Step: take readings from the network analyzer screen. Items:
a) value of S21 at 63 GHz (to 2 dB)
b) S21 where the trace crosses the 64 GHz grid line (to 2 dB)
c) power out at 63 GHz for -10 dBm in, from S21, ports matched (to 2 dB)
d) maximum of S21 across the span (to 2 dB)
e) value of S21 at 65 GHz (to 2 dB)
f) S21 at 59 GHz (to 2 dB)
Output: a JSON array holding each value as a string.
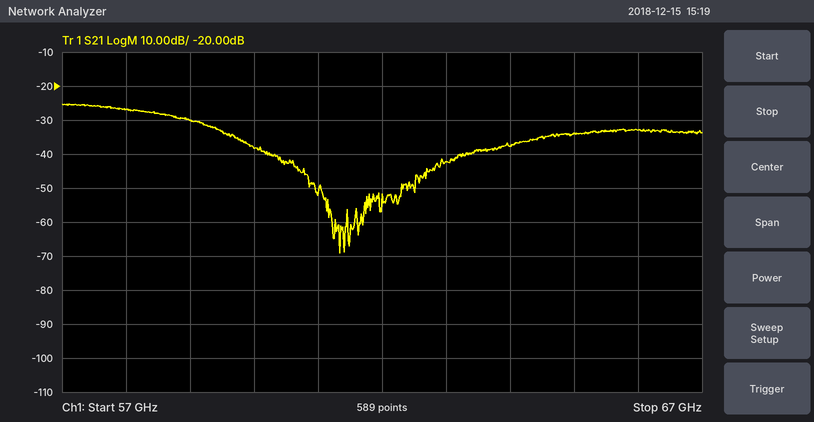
["-42 dB", "-38 dB", "-52 dBm", "-26 dB", "-34 dB", "-30 dB"]
